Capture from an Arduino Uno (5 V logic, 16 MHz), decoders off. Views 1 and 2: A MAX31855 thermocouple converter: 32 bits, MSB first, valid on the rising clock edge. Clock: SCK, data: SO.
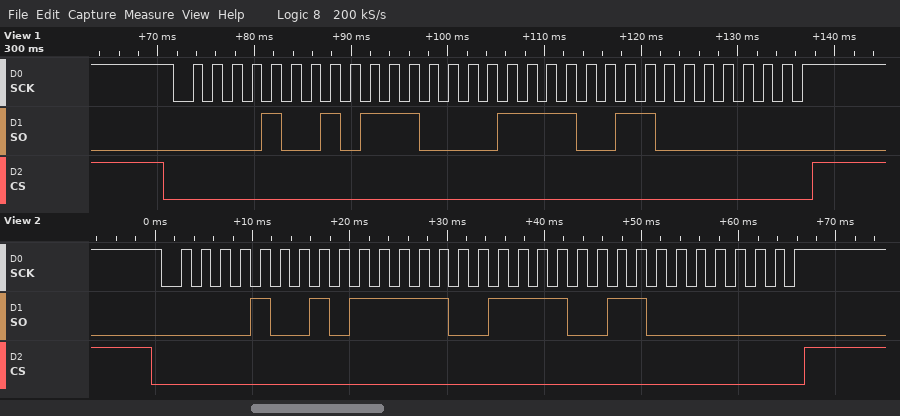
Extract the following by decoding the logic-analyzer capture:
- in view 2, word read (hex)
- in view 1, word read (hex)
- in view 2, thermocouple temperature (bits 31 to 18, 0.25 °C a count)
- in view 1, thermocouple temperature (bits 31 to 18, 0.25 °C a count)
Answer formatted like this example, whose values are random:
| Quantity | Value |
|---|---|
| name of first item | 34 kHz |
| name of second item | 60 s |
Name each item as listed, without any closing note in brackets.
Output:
| Quantity | Value |
|---|---|
| in view 2, word read | 0x097CF300 |
| in view 1, word read | 0x0970F300 |
| in view 2, thermocouple temperature | 151.75 °C |
| in view 1, thermocouple temperature | 151.00 °C |
